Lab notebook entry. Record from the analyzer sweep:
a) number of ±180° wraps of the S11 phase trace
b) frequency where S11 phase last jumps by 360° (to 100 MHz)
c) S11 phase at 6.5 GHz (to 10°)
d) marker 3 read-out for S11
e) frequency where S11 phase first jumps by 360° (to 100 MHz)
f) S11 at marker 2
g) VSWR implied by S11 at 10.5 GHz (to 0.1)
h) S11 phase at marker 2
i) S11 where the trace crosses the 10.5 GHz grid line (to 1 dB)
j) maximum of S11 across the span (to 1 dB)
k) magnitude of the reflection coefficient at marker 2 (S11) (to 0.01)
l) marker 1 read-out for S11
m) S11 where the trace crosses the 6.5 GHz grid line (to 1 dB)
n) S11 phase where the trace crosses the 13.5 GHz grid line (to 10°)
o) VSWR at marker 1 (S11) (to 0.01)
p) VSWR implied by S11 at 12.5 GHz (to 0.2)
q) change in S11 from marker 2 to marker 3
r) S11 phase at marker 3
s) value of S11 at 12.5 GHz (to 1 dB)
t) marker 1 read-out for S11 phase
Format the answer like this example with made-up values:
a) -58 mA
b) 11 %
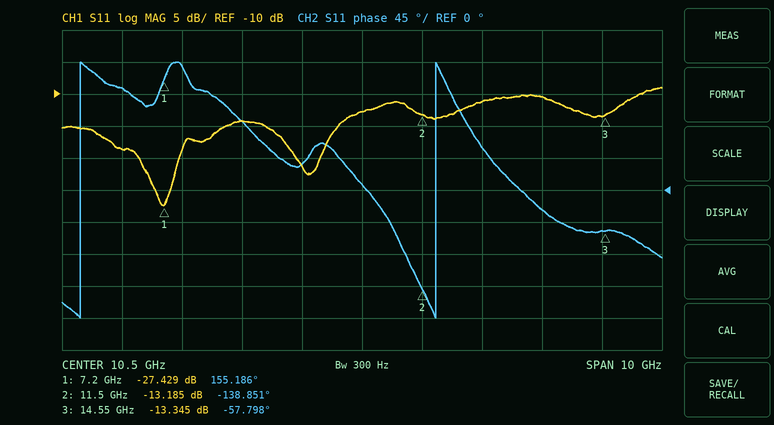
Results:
a) 2
b) 11.7 GHz
c) 140°
d) -13.345 dB
e) 5.8 GHz
f) -13.185 dB
g) 1.6
h) -138.851°
i) -13 dB
j) -9 dB
k) 0.22
l) -27.429 dB
m) -19 dB
n) -30°
o) 1.09
p) 1.8
q) -0.160 dB
r) -57.798°
s) -11 dB
t) 155.186°
